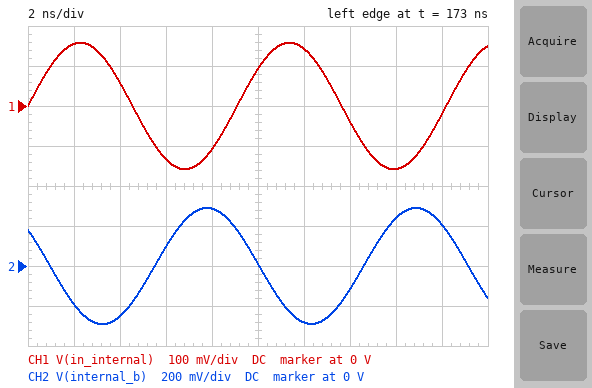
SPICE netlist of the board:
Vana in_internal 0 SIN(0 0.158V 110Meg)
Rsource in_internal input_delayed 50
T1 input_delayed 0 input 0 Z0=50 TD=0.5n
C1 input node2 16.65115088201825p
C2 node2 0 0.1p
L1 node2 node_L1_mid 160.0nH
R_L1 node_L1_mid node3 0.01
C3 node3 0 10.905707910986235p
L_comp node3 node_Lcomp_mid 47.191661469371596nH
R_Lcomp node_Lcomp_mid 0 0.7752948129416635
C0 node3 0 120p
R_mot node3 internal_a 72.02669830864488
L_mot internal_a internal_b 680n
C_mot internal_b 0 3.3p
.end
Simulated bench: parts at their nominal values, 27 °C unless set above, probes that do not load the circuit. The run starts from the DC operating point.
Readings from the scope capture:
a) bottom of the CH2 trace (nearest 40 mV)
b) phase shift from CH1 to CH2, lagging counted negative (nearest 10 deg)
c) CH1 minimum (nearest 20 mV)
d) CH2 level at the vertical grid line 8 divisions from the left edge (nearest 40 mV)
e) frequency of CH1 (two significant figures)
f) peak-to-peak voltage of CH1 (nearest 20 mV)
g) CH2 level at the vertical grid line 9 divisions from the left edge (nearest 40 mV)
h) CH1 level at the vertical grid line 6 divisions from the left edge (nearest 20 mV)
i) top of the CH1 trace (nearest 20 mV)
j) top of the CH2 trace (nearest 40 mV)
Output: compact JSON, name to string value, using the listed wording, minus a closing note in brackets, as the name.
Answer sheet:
{"bottom of the CH2 trace": "-280 mV", "phase shift from CH1 to CH2, lagging counted negative": "140 deg", "CH1 minimum": "-160 mV", "CH2 level at the vertical grid line 8 divisions from the left edge": "240 mV", "frequency of CH1": "110 MHz", "peak-to-peak voltage of CH1": "320 mV", "CH2 level at the vertical grid line 9 divisions from the left edge": "200 mV", "CH1 level at the vertical grid line 6 divisions from the left edge": "140 mV", "top of the CH1 trace": "160 mV", "top of the CH2 trace": "280 mV"}
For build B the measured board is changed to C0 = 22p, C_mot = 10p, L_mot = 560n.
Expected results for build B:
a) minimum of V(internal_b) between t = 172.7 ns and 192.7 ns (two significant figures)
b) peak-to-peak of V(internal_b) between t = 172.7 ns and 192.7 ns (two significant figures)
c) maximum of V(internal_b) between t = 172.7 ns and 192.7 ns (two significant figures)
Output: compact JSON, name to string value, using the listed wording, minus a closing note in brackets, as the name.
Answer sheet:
{"minimum of V(internal_b) between t = 172.7 ns and 192.7 ns": "-61 mV", "peak-to-peak of V(internal_b) between t = 172.7 ns and 192.7 ns": "120 mV", "maximum of V(internal_b) between t = 172.7 ns and 192.7 ns": "61 mV"}
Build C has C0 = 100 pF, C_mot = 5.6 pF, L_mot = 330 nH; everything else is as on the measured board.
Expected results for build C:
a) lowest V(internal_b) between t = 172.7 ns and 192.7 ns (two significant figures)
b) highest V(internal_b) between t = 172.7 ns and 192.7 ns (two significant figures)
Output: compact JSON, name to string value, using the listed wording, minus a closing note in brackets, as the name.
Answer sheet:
{"lowest V(internal_b) between t = 172.7 ns and 192.7 ns": "-180 mV", "highest V(internal_b) between t = 172.7 ns and 192.7 ns": "180 mV"}
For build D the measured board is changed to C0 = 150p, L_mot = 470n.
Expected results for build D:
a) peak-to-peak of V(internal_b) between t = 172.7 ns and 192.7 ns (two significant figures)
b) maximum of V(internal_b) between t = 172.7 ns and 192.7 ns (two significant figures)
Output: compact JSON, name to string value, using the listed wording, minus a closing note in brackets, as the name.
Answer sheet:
{"peak-to-peak of V(internal_b) between t = 172.7 ns and 192.7 ns": "230 mV", "maximum of V(internal_b) between t = 172.7 ns and 192.7 ns": "110 mV"}
